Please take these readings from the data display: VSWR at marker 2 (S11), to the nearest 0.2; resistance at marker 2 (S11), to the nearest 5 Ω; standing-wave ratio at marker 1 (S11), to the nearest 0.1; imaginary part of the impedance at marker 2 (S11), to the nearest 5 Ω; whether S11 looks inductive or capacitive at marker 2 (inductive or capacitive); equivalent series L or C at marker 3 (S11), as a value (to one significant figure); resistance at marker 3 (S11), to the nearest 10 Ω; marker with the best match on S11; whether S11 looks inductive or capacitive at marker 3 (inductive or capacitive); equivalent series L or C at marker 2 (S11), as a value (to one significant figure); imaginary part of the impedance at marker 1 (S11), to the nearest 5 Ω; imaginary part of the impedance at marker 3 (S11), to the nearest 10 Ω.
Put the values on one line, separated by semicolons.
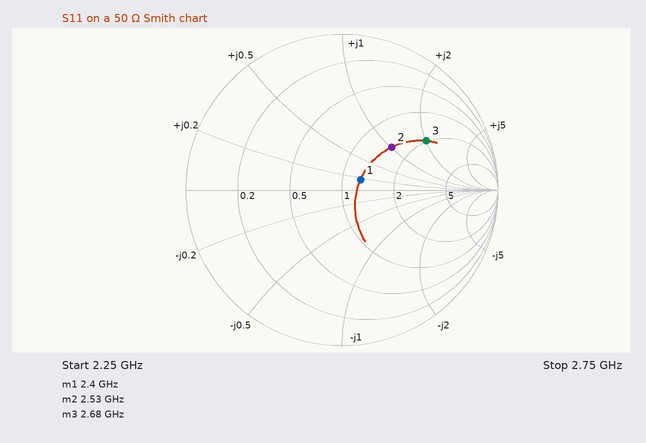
2.4; 75 Ω; 1.3; +50 Ω; inductive; 6 nH; 100 Ω; marker 1; inductive; 3 nH; +10 Ω; +100 Ω
